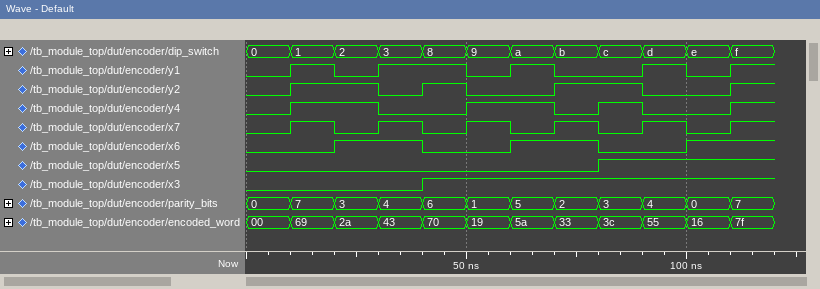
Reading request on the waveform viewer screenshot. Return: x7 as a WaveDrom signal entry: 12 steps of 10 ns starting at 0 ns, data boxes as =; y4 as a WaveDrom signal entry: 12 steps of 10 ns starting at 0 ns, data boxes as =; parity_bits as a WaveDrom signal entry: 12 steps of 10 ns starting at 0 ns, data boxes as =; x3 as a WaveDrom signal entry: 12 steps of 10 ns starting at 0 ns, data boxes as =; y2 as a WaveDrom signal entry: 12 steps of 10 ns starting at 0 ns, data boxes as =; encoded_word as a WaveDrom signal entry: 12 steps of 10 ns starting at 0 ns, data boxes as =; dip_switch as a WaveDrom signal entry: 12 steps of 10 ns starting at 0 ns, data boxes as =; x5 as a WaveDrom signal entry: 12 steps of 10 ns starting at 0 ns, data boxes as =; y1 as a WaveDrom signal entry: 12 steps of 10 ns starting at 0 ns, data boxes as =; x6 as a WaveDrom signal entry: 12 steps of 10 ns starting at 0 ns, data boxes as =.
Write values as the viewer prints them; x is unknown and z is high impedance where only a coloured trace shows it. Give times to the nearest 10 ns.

{name: 'x7', wave: '010101010101'}
{name: 'y4', wave: '01.0.1.010.1'}
{name: 'parity_bits', wave: '============', data: '0 7 3 4 6 1 5 2 3 4 0 7'}
{name: 'x3', wave: '0...1.......'}
{name: 'y2', wave: '01.010.1.0.1'}
{name: 'encoded_word', wave: '============', data: '00 69 2a 43 70 19 5a 33 3c 55 16 7f'}
{name: 'dip_switch', wave: '============', data: '0 1 2 3 8 9 a b c d e f'}
{name: 'x5', wave: '0.......1...'}
{name: 'y1', wave: '0101.010.101'}
{name: 'x6', wave: '0.1.0.1.0.1.'}
